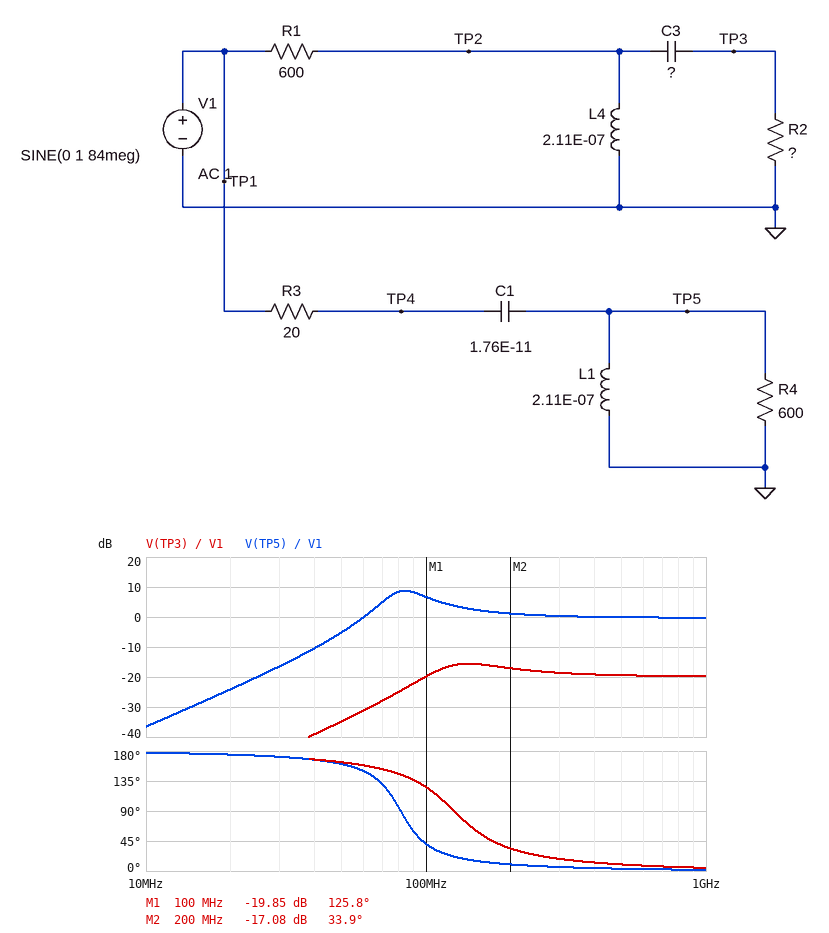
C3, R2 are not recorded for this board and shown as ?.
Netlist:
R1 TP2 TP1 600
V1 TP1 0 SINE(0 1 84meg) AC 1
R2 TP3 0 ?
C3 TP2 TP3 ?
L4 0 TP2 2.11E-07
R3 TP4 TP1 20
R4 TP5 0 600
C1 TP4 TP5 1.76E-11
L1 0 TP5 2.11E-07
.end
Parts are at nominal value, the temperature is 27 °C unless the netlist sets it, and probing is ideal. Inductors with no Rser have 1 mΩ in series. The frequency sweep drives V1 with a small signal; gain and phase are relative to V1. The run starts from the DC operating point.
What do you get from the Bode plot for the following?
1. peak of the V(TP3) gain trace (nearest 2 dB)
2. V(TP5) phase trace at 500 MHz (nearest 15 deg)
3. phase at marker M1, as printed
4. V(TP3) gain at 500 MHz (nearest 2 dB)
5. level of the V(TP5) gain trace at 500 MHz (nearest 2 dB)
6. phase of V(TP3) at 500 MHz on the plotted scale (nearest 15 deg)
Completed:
-16 dB
0 deg
125.8 deg
-20 dB
0 dB
15 deg
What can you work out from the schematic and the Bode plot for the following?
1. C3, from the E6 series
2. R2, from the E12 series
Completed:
6.8 pF
68 Ω
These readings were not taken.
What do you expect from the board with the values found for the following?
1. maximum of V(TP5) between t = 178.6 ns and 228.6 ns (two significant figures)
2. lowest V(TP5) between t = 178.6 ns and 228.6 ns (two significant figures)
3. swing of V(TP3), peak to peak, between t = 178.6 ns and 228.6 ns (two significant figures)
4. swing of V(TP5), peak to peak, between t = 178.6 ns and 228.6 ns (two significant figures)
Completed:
2.7 V
-2.7 V
130 mV
5.5 V
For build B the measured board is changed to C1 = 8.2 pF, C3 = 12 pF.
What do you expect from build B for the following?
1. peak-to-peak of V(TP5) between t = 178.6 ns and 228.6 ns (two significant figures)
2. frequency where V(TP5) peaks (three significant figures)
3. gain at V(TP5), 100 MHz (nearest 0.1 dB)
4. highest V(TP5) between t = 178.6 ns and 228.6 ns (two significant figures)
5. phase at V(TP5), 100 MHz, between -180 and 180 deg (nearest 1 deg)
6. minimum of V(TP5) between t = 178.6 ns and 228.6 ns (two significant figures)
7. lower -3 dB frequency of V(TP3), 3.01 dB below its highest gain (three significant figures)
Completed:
1.7 V
124 MHz
3.9 dB
840 mV
132 deg
-840 mV
79.8 MHz
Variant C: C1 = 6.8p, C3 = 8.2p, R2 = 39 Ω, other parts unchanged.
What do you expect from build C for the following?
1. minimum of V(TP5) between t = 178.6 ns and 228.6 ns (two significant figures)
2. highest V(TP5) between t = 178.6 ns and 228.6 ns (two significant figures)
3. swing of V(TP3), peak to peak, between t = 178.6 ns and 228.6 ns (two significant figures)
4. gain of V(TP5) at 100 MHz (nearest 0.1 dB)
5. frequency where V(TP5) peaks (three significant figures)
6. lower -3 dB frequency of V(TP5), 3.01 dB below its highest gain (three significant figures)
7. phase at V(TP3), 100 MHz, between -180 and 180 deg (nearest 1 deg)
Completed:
-620 mV
620 mV
100 mV
0.8 dB
136 MHz
114 MHz
123 deg
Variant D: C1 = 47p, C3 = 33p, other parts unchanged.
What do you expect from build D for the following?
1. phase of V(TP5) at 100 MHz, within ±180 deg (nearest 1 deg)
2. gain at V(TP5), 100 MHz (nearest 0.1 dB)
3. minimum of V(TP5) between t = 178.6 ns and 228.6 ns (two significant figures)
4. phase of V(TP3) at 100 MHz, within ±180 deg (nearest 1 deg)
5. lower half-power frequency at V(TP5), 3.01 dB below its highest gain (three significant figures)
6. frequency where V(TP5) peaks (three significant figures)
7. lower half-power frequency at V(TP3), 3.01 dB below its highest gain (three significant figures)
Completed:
15 deg
1.9 dB
-1.4 V
38 deg
43.4 MHz
51.9 MHz
48.5 MHz
